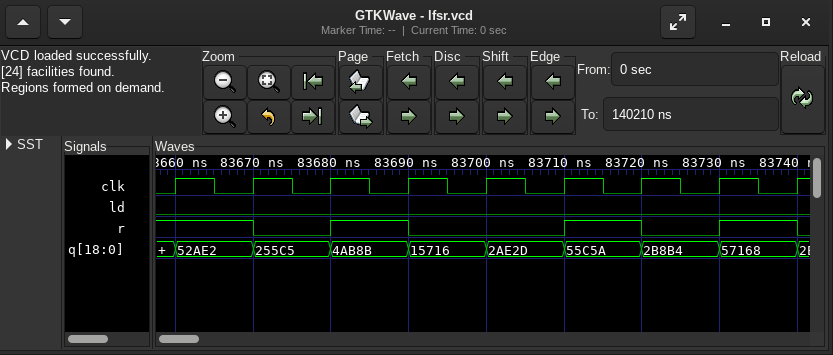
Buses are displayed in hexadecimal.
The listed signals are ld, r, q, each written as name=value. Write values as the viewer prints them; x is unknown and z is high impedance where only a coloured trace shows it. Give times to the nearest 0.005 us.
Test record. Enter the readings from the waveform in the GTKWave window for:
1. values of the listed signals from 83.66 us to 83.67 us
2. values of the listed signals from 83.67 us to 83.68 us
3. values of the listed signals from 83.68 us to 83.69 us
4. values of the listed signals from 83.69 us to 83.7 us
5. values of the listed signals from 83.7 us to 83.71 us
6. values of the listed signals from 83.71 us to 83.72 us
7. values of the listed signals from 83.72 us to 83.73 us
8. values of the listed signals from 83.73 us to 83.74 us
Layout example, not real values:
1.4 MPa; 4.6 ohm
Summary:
ld=0, r=1, q=52AE2; ld=0, r=0, q=255C5; ld=0, r=1, q=4AB8B; ld=0, r=0, q=15716; ld=0, r=0, q=2AE2D; ld=0, r=1, q=55C5A; ld=0, r=0, q=2B8B4; ld=0, r=1, q=57168
